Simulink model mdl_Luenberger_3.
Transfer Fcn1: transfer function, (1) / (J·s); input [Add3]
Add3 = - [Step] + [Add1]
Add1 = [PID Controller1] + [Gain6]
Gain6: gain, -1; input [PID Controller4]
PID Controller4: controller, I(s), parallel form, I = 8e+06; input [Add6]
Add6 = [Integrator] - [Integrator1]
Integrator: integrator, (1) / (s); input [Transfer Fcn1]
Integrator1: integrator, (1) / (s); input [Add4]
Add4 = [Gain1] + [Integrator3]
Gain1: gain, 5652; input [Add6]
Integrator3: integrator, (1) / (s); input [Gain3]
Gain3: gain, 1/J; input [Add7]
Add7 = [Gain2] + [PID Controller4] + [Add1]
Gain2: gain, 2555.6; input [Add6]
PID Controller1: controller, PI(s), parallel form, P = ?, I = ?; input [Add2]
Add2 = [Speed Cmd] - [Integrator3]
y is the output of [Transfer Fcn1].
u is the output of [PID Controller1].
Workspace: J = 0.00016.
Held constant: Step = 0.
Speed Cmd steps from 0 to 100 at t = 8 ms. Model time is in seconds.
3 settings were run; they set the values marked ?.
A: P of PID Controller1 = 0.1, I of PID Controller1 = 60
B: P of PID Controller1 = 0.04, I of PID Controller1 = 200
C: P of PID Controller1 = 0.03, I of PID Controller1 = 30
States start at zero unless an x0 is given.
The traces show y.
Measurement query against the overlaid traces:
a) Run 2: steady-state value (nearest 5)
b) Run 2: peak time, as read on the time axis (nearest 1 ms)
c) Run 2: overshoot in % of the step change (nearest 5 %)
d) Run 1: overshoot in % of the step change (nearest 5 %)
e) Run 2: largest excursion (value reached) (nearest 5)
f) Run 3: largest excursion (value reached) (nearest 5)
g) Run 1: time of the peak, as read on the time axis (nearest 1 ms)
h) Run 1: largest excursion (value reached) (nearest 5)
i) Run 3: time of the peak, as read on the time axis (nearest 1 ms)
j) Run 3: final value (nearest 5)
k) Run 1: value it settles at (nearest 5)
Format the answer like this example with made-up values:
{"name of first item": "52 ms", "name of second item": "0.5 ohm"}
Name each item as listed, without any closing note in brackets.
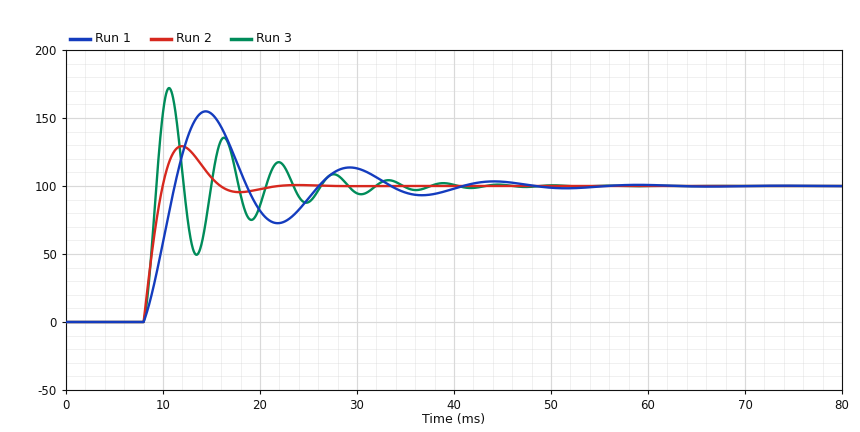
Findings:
{"Run 2: steady-state value": "100", "Run 2: peak time, as read on the time axis": "12 ms", "Run 2: overshoot in % of the step change": "30 %", "Run 1: overshoot in % of the step change": "55 %", "Run 2: largest excursion (value reached)": "130", "Run 3: largest excursion (value reached)": "170", "Run 1: time of the peak, as read on the time axis": "14 ms", "Run 1: largest excursion (value reached)": "155", "Run 3: time of the peak, as read on the time axis": "11 ms", "Run 3: final value": "100", "Run 1: value it settles at": "100"}
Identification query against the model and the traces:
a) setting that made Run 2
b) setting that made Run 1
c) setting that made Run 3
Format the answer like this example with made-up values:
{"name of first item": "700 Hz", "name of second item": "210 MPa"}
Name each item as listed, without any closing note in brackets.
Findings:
{"setting that made Run 2": "A", "setting that made Run 1": "C", "setting that made Run 3": "B"}
